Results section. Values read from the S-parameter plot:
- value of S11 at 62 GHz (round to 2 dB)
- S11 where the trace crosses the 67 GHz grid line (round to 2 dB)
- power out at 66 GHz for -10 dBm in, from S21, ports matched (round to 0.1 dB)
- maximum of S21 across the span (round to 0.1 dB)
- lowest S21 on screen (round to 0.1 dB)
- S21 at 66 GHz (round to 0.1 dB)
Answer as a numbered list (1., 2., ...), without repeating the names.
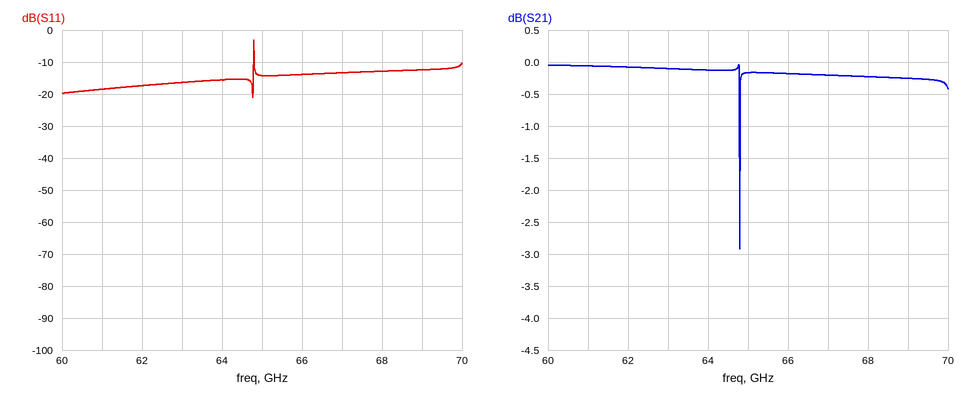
1. -18 dB
2. -14 dB
3. -10.2 dBm
4. 0.0 dB
5. -2.9 dB
6. -0.2 dB
